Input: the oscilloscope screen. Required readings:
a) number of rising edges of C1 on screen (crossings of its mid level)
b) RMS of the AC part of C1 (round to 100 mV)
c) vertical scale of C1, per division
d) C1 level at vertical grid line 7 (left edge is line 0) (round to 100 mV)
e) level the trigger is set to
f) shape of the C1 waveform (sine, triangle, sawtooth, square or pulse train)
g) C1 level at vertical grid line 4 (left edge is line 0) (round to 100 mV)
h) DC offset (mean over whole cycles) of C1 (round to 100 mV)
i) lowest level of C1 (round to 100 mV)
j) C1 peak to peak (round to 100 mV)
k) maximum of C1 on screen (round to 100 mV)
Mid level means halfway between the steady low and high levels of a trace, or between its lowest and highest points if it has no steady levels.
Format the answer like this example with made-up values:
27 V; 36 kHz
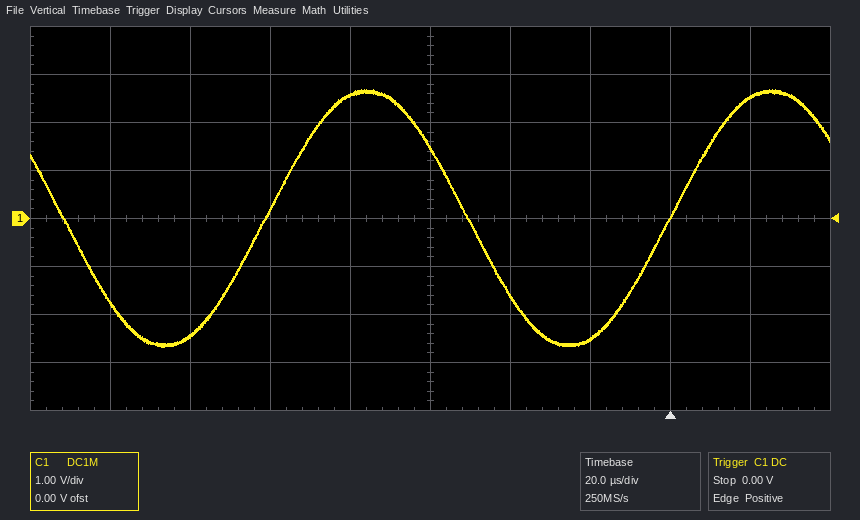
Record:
2; 1.9 V; 1 V; -2.5 V; 0.00 V; sine; 2.6 V; 0.0 V; -2.7 V; 5.4 V; 2.7 V
